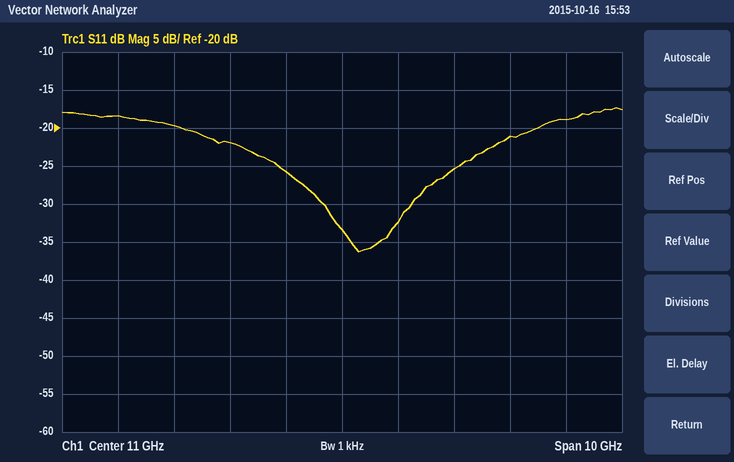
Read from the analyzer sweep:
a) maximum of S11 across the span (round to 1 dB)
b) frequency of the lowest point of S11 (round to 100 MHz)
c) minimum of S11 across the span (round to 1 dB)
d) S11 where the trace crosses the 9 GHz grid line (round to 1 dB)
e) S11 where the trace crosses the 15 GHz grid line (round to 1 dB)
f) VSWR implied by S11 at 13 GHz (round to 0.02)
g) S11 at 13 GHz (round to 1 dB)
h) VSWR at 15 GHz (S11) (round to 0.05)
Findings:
-17 dB
11.3 GHz
-36 dB
-22 dB
-19 dB
1.12
-25 dB
1.25
